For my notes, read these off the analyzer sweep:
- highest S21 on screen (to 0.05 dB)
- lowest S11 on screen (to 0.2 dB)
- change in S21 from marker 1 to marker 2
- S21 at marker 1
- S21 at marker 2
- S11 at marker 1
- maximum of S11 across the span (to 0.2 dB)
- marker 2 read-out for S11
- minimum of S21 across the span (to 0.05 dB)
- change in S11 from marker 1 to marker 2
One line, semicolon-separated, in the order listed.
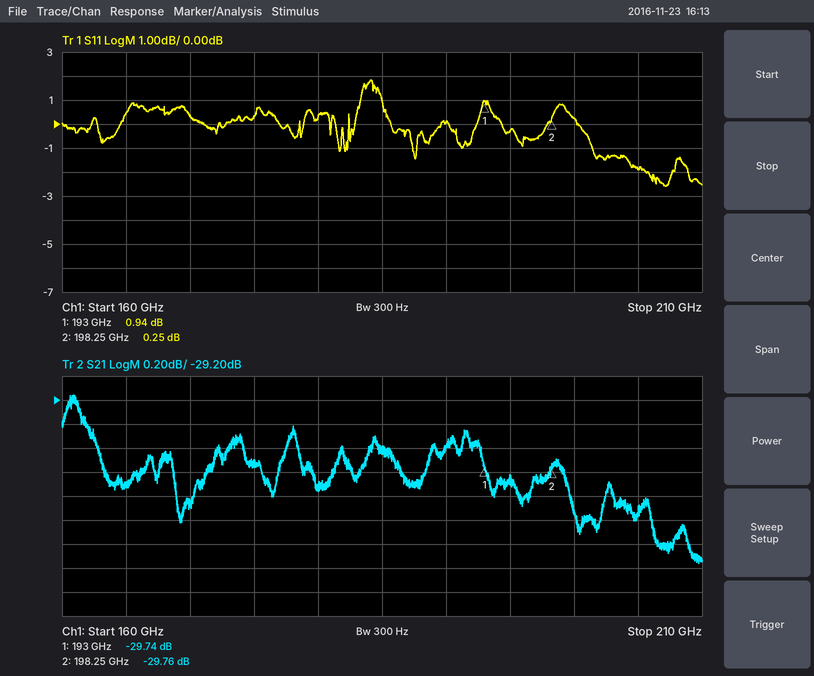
-29.15 dB; -2.6 dB; -0.02 dB; -29.74 dB; -29.76 dB; 0.94 dB; 1.8 dB; 0.25 dB; -30.55 dB; -0.69 dB
